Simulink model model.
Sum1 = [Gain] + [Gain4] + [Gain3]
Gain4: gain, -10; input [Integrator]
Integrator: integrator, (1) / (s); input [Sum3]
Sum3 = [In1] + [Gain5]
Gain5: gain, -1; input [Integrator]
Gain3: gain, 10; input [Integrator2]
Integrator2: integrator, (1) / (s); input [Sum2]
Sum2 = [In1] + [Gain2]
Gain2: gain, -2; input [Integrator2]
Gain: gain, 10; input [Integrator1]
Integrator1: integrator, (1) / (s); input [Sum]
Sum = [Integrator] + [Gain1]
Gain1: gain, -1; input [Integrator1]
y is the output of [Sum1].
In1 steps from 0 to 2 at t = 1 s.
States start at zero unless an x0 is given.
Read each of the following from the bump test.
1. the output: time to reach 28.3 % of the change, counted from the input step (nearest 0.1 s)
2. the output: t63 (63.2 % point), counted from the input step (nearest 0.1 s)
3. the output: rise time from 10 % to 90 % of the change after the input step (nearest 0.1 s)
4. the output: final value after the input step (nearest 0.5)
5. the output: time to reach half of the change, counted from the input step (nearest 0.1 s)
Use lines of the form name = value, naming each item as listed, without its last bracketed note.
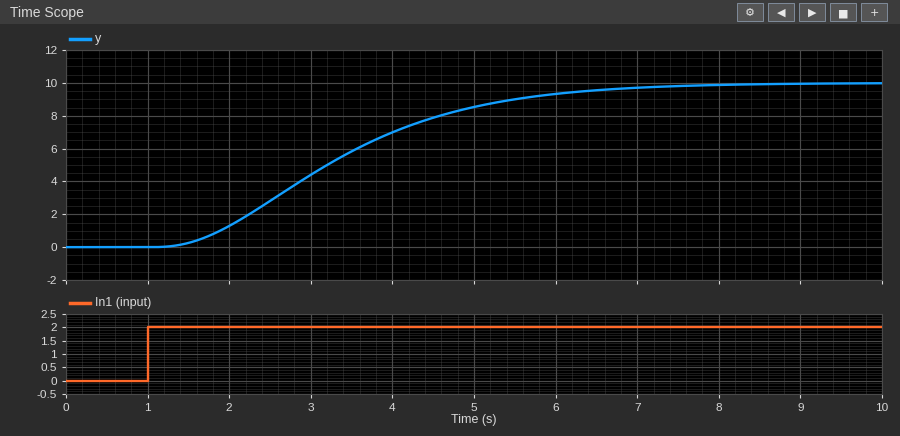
the output: time to reach 28.3 % of the change, counted from the input step = 1.5 s
the output: t63 (63.2 % point), counted from the input step = 2.7 s
the output: rise time from 10 % to 90 % of the change after the input step = 3.6 s
the output: final value after the input step = 10.0
the output: time to reach half of the change, counted from the input step = 2.2 s
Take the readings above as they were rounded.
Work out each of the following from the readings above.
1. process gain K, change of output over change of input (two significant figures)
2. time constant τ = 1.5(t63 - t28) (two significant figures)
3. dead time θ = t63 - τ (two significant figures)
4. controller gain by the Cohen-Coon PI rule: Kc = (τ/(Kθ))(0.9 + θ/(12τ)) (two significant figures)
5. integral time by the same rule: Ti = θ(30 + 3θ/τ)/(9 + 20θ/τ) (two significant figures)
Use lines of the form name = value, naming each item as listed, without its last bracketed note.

process gain K, change of output over change of input = 5.0
time constant τ = 1.5(t63 - t28) = 1.8 s
dead time θ = t63 - τ = 0.90 s
controller gain by the Cohen-Coon PI rule: Kc = (τ/(Kθ))(0.9 + θ/(12τ)) = 0.38
integral time by the same rule: Ti = θ(30 + 3θ/τ)/(9 + 20θ/τ) = 1.5 s
